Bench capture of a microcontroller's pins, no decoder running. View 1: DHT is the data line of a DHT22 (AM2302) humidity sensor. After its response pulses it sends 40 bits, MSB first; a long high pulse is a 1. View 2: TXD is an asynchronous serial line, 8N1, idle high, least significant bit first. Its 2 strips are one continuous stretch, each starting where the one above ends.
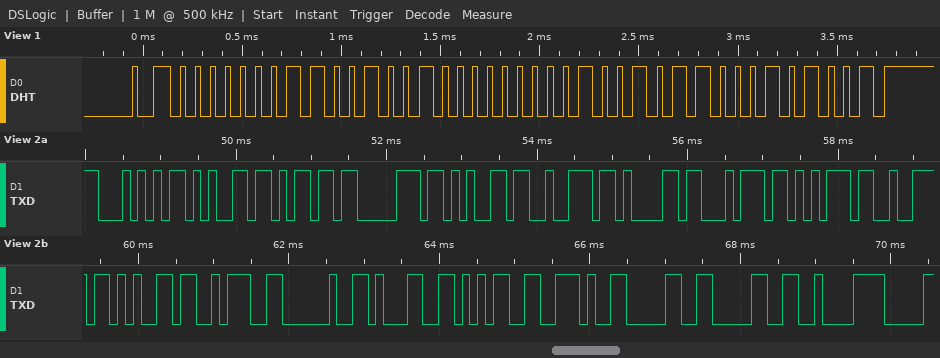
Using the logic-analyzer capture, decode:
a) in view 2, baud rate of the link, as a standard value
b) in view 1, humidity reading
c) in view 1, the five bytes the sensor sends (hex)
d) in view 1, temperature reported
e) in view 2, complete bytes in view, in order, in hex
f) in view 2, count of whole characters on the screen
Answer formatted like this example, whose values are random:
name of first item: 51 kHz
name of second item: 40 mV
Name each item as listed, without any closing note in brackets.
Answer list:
in view 2, baud rate of the link, as a standard value: 9600 baud
in view 1, humidity reading: 40.2 %
in view 1, the five bytes the sensor sends: 01 92 00 96 29
in view 1, temperature reported: 15.0 °C
in view 2, complete bytes in view, in order, in hex: 0x54 0x65 0x6D 0x70 0x65 0x72 0x61 0x74 0x75 0x72 0x65 0x3A 0x20 0x31 0x35 0x2E 0x30 0x30 0xC2
in view 2, count of whole characters on the screen: 19
